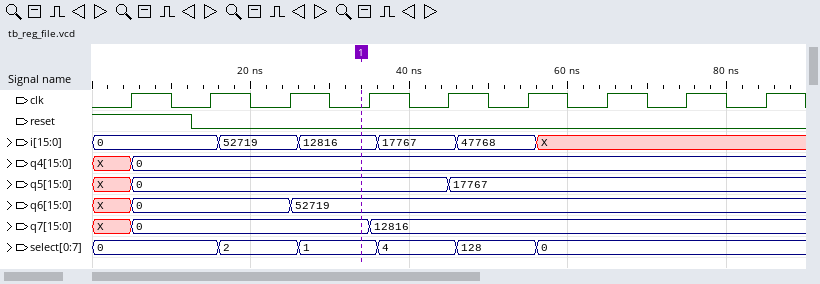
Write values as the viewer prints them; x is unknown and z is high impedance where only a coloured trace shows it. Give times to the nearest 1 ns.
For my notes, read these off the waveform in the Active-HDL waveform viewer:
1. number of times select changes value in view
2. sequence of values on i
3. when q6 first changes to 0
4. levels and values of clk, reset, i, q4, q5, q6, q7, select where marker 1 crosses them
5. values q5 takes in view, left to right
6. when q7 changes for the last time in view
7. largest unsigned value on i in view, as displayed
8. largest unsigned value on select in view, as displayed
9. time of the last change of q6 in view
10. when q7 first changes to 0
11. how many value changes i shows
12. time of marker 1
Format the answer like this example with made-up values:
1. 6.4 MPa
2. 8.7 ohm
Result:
1. 5
2. 0, 52719, 12816, 17767, 47768, X
3. 5 ns
4. clk=0, reset=0, i=12816, q4=0, q5=0, q6=52719, q7=0, select=1
5. X, 0, 17767
6. 35 ns
7. 52719
8. 128
9. 25 ns
10. 5 ns
11. 5
12. 34 ns
